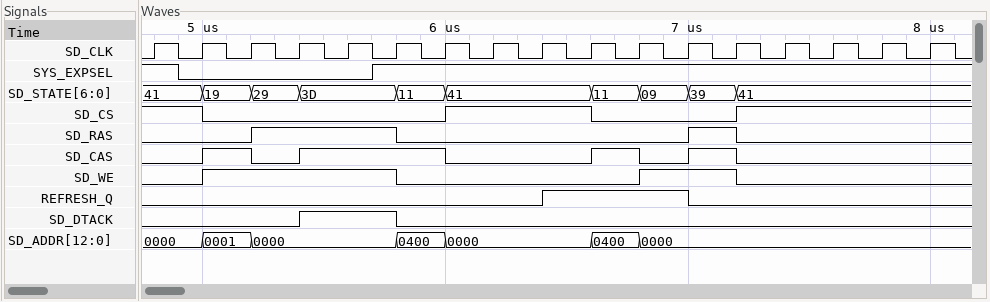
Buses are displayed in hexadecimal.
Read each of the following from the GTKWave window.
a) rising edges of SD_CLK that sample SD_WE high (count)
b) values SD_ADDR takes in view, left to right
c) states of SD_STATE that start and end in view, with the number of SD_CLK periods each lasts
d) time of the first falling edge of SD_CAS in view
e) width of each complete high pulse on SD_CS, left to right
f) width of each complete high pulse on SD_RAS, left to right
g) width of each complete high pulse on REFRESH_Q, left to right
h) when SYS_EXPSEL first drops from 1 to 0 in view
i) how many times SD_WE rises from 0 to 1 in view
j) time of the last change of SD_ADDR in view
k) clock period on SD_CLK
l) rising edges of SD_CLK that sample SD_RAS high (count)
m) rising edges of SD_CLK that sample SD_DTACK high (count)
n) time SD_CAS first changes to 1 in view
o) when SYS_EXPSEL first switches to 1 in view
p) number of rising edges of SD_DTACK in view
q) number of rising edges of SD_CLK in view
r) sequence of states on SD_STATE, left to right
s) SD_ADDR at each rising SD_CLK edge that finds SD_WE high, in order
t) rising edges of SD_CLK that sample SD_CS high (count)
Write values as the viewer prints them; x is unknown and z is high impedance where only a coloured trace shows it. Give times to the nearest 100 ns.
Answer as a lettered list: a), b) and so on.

a) 6
b) 0000, 0001, 0000, 0400, 0000, 0400, 0000
c) 19: 1, 29: 1, 3D: 2, 11: 1, 41: 3, 11: 1, 09: 1, 39: 1
d) 5200 ns
e) 600 ns
f) 600 ns, 200 ns
g) 600 ns
h) 4900 ns
i) 2
j) 6800 ns
k) 200 ns
l) 4
m) 2
n) 5000 ns
o) 5700 ns
p) 1
q) 17
r) 41, 19, 29, 3D, 11, 41, 11, 09, 39, 41
s) 0001, 0000, 0000, 0000, 0000, 0000
t) 9
